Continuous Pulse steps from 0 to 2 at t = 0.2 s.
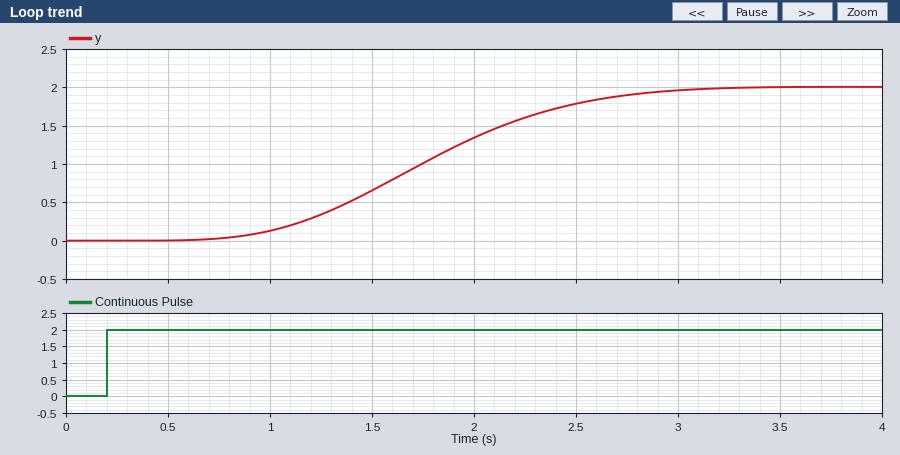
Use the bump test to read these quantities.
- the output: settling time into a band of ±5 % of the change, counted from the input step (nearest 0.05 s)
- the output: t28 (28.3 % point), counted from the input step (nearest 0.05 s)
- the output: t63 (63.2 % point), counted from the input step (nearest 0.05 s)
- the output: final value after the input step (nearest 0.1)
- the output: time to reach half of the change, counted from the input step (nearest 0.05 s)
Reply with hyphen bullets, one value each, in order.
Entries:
- 2.55 s
- 1.25 s
- 1.75 s
- 2.0
- 1.55 s
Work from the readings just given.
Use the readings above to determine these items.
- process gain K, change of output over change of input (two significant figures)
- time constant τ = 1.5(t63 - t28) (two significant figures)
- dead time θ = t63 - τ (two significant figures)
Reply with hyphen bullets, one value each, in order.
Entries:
- 1.0
- 0.75 s
- 1.0 s
